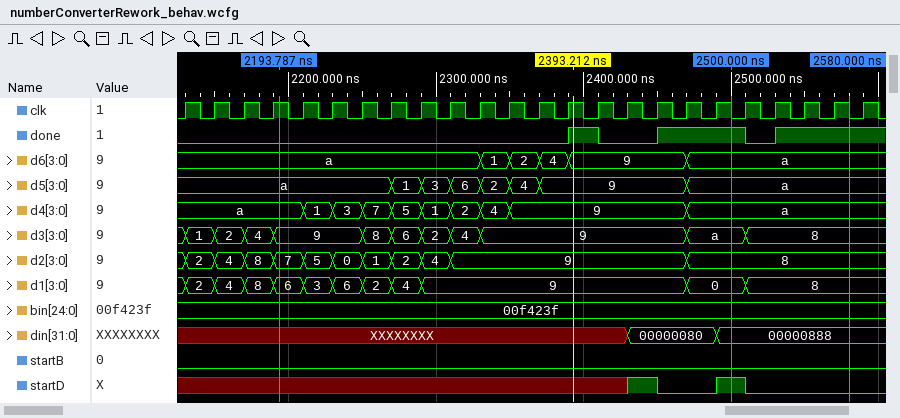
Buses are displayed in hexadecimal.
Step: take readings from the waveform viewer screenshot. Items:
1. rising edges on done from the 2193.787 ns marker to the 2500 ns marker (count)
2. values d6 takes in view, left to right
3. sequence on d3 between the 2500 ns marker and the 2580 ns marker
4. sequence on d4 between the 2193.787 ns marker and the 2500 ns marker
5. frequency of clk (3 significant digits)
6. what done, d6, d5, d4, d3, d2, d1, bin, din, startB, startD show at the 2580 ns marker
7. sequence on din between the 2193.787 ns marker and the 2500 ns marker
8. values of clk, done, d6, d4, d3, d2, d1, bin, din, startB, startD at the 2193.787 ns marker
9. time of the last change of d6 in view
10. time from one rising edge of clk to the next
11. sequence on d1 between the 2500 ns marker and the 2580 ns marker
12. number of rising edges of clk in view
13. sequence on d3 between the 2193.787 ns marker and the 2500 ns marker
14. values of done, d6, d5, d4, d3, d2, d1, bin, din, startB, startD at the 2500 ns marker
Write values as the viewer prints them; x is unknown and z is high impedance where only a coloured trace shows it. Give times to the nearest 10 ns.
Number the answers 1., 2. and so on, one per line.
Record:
1. 2
2. a, 1, 2, 4, 9, a
3. a, 8
4. a, 1, 3, 7, 5, 1, 2, 4, 9, a
5. 50.0 MHz
6. done=1, d6=a, d5=a, d4=a, d3=8, d2=8, d1=8, bin=00f423f, din=00000888, startB=0, startD=0
7. XXXXXXXX, 00000080, 00000888
8. clk=1, done=0, d6=a, d4=a, d3=9, d2=7, d1=6, bin=00f423f, din=XXXXXXXX, startB=0, startD=x
9. 2470 ns
10. 20 ns
11. 0, 8
12. 24
13. 9, 8, 6, 2, 4, 9, a
14. done=1, d6=a, d5=a, d4=a, d3=a, d2=8, d1=0, bin=00f423f, din=00000888, startB=0, startD=1
